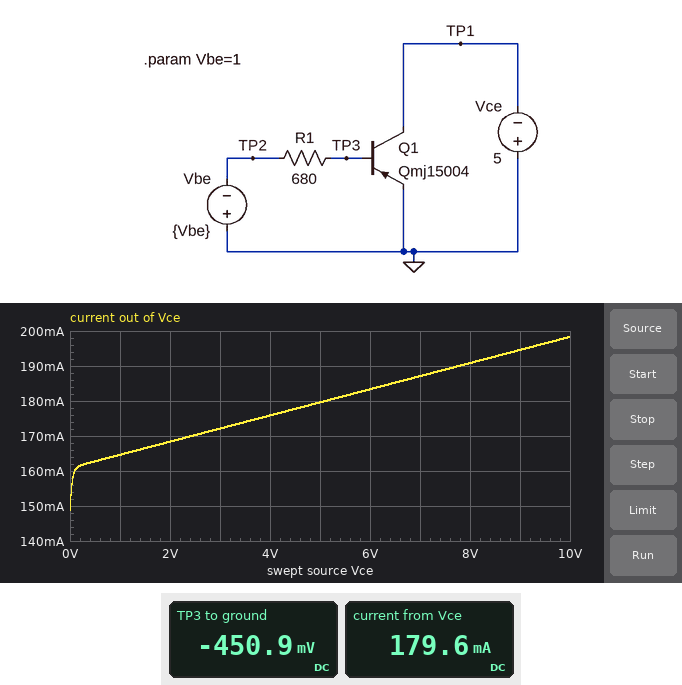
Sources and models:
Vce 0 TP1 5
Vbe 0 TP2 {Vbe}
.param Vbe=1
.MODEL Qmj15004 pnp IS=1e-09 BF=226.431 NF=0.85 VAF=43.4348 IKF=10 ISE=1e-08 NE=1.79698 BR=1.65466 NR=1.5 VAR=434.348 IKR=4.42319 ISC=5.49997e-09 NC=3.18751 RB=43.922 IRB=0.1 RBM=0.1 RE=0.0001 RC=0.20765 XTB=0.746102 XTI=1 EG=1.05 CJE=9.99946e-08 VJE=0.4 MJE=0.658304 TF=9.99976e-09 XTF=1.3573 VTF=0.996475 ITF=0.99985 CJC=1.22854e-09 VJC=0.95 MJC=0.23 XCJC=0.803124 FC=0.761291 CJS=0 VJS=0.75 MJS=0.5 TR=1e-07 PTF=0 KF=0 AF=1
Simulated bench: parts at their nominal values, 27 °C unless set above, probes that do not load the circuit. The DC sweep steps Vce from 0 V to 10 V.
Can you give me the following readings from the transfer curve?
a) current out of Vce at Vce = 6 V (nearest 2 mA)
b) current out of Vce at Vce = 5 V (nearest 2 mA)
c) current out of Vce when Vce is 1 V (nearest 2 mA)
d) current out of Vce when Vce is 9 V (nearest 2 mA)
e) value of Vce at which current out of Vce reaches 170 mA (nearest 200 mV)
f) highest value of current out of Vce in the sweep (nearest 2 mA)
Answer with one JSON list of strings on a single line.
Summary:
["184 mA", "180 mA", "164 mA", "194 mA", "2.4 V", "198 mA"]
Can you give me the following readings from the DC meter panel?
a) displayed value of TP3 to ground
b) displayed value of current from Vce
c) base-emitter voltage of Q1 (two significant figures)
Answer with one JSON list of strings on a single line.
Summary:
["-450.9 mV", "179.6 mA", "-450 mV"]
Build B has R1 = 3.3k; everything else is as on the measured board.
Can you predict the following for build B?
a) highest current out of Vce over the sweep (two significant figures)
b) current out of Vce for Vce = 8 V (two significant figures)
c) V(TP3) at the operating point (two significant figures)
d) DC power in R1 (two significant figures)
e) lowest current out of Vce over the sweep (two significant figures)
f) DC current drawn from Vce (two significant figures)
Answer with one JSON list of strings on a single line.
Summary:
["41 mA", "39 mA", "-390 mV", "110 µW", "31 mA", "37 mA"]
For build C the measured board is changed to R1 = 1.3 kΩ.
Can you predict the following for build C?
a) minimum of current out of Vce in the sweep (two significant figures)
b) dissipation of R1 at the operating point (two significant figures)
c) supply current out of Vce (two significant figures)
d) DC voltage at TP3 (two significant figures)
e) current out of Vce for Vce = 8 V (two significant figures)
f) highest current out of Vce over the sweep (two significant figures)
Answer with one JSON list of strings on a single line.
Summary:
["80 mA", "260 µW", "96 mA", "-420 mV", "100 mA", "110 mA"]
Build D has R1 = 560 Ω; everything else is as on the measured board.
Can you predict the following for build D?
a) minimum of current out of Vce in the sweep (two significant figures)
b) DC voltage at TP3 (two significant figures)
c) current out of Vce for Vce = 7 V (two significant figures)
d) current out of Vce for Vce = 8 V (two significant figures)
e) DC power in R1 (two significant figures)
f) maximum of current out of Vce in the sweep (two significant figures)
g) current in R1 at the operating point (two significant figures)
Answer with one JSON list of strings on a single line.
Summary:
["180 mA", "-460 mV", "220 mA", "230 mA", "520 µW", "240 mA", "960 µA"]
